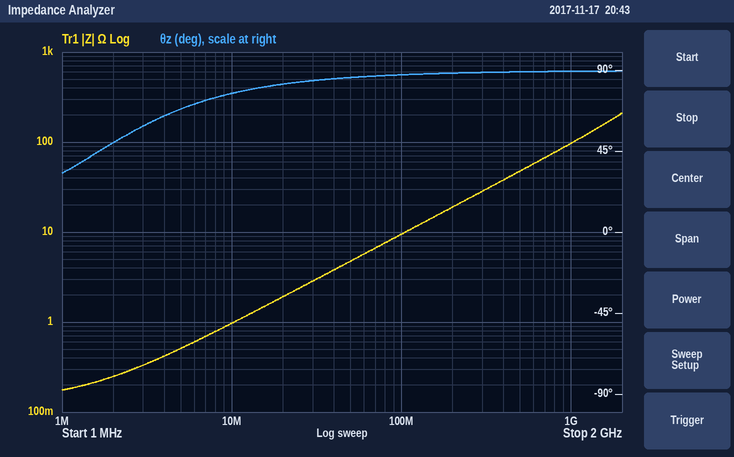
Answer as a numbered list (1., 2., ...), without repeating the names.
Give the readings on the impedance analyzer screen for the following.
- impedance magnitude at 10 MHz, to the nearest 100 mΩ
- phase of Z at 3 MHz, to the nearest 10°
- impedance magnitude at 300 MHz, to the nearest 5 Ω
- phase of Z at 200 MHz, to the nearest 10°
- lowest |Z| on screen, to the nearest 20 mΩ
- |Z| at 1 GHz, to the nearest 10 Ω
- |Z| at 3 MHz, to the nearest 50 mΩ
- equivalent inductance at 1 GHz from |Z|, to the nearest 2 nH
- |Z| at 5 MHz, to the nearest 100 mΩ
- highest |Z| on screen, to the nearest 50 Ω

1. 1.0 Ω
2. 60°
3. 30 Ω
4. 90°
5. 180 mΩ
6. 100 Ω
7. 350 mΩ
8. 16 nH
9. 500 mΩ
10. 200 Ω
